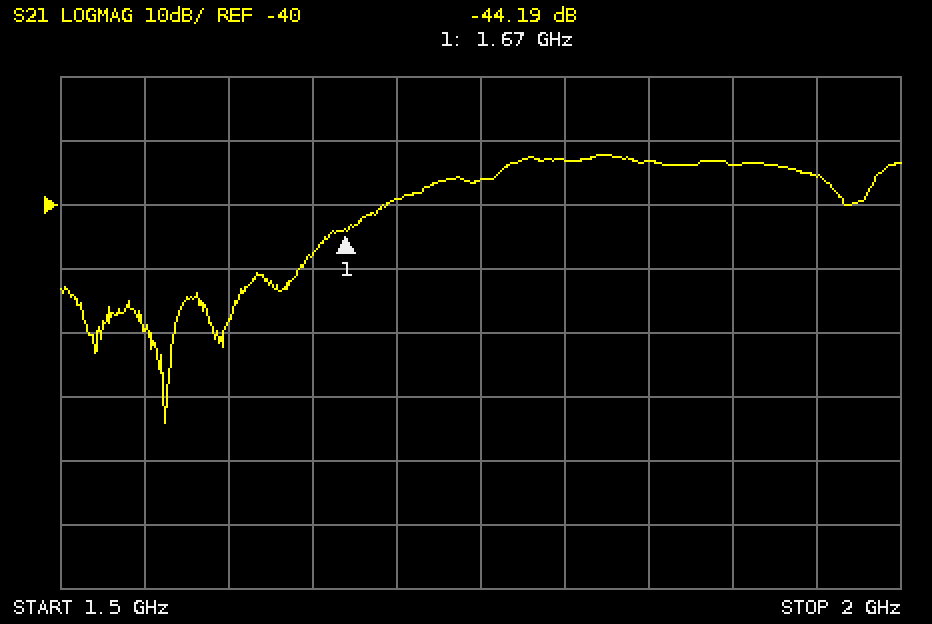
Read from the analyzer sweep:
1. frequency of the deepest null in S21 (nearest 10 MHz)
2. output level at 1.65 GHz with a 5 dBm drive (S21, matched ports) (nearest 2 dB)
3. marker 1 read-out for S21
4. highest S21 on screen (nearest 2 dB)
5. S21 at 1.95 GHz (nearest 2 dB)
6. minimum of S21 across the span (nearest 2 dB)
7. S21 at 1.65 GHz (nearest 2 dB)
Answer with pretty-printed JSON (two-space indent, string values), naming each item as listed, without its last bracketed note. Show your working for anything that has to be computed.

{
  "frequency of the deepest null in S21": "1.56 GHz",
  "output level at 1.65 GHz with a 5 dBm drive (S21, matched ports)": "5 dBm + (-48 dB) = -42 dBm",
  "marker 1 read-out for S21": "-44.19 dB",
  "highest S21 on screen": "-32 dB",
  "S21 at 1.95 GHz": "-36 dB",
  "minimum of S21 across the span": "-74 dB",
  "S21 at 1.65 GHz": "-48 dB"
}
